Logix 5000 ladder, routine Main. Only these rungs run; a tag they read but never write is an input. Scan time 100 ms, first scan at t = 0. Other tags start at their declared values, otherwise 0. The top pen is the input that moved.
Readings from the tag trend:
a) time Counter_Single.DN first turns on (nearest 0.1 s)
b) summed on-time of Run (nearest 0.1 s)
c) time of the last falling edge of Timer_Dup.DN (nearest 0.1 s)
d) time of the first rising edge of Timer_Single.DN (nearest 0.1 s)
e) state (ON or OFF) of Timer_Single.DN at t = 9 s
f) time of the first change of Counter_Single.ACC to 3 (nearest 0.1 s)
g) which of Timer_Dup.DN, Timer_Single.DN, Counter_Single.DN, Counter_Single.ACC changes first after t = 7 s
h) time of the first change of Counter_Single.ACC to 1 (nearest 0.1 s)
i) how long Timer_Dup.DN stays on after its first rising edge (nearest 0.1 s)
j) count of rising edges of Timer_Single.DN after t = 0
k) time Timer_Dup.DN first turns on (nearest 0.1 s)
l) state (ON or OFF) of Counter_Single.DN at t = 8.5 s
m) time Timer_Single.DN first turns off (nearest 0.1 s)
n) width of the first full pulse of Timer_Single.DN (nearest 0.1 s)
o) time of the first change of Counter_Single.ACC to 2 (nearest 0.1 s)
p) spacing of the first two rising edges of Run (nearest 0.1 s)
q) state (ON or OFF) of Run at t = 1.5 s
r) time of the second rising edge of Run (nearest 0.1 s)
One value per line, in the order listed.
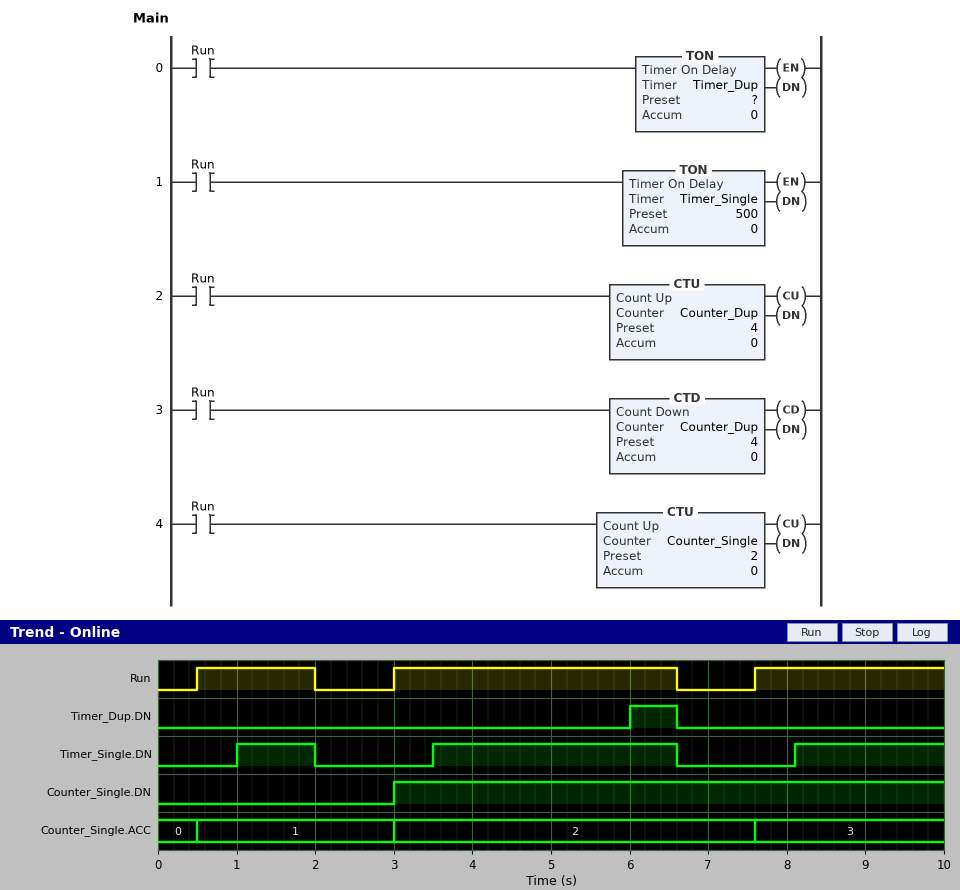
3.0 s
7.5 s
6.6 s
1.0 s
ON
7.6 s
Counter_Single.ACC
0.5 s
0.6 s
3
6.0 s
ON
2.0 s
1.0 s
3.0 s
2.5 s
ON
3.0 s
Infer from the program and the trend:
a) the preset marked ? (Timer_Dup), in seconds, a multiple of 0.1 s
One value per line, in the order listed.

3.0 s
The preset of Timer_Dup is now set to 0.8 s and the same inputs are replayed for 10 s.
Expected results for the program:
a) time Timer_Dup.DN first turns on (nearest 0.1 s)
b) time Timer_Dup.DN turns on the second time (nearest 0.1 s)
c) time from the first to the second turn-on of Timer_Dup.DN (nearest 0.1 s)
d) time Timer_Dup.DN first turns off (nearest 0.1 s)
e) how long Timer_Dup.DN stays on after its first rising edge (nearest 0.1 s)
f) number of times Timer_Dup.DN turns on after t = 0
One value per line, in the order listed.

1.3 s
3.8 s
2.5 s
2.0 s
0.7 s
3
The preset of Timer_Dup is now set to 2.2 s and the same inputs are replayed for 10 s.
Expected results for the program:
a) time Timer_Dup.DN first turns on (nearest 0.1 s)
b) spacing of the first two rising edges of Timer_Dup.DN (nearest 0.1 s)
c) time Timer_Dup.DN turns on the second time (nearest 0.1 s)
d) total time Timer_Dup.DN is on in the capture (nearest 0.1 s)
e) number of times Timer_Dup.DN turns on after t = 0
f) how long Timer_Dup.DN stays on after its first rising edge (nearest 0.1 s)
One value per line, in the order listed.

5.2 s
4.6 s
9.8 s
1.6 s
2
1.4 s
